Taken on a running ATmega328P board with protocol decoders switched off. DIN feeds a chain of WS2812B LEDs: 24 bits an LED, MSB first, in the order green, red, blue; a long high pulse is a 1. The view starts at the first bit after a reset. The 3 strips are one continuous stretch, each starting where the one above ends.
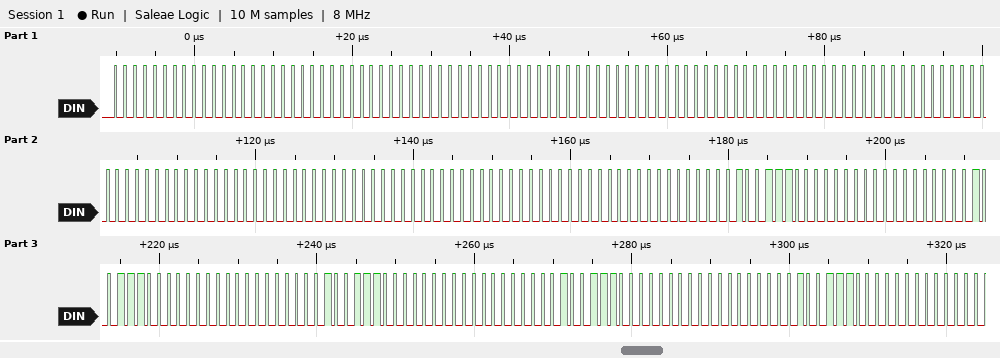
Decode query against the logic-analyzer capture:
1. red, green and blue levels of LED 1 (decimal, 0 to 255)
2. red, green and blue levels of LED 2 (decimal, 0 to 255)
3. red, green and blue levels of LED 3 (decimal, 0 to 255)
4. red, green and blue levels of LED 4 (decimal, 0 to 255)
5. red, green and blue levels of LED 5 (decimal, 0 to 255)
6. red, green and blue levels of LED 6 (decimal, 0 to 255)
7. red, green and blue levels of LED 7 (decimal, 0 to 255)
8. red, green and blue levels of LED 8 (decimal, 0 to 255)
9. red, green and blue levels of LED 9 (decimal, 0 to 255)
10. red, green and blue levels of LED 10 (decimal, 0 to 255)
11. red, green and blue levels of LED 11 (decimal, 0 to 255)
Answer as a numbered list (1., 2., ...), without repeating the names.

1. 0, 0, 0
2. 0, 0, 0
3. 0, 0, 0
4. 0, 0, 0
5. 0, 0, 0
6. 0, 0, 0
7. 78, 0, 0
8. 78, 0, 0
9. 78, 0, 0
10. 78, 0, 0
11. 78, 0, 0
